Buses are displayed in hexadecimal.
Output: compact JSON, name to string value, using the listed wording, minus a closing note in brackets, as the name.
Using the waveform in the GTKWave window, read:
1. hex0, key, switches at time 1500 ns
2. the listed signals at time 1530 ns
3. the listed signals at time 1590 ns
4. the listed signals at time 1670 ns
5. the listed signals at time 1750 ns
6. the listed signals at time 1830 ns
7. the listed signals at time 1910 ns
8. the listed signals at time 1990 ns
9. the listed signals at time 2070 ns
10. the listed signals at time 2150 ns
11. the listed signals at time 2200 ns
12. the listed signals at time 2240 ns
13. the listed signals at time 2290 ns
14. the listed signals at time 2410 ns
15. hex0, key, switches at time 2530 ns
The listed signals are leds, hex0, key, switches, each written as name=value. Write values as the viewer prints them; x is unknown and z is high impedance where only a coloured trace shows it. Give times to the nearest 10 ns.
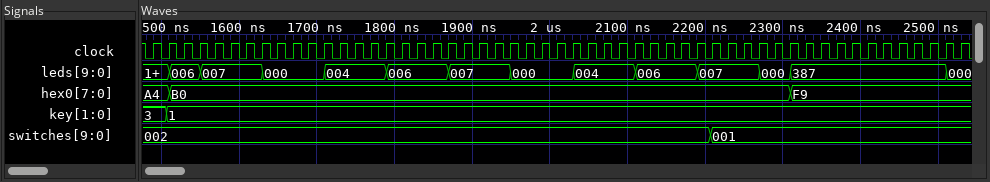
{"hex0, key, switches at time 1500 ns": "hex0=A4, key=3, switches=002", "the listed signals at time 1530 ns": "leds=006, hex0=B0, key=1, switches=002", "the listed signals at time 1590 ns": "leds=007, hex0=B0, key=1, switches=002", "the listed signals at time 1670 ns": "leds=000, hex0=B0, key=1, switches=002", "the listed signals at time 1750 ns": "leds=004, hex0=B0, key=1, switches=002", "the listed signals at time 1830 ns": "leds=006, hex0=B0, key=1, switches=002", "the listed signals at time 1910 ns": "leds=007, hex0=B0, key=1, switches=002", "the listed signals at time 1990 ns": "leds=000, hex0=B0, key=1, switches=002", "the listed signals at time 2070 ns": "leds=004, hex0=B0, key=1, switches=002", "the listed signals at time 2150 ns": "leds=006, hex0=B0, key=1, switches=002", "the listed signals at time 2200 ns": "leds=007, hex0=B0, key=1, switches=002", "the listed signals at time 2240 ns": "leds=007, hex0=B0, key=1, switches=001", "the listed signals at time 2290 ns": "leds=000, hex0=B0, key=1, switches=001", "the listed signals at time 2410 ns": "leds=387, hex0=F9, key=1, switches=001", "hex0, key, switches at time 2530 ns": "hex0=F9, key=1, switches=001"}
